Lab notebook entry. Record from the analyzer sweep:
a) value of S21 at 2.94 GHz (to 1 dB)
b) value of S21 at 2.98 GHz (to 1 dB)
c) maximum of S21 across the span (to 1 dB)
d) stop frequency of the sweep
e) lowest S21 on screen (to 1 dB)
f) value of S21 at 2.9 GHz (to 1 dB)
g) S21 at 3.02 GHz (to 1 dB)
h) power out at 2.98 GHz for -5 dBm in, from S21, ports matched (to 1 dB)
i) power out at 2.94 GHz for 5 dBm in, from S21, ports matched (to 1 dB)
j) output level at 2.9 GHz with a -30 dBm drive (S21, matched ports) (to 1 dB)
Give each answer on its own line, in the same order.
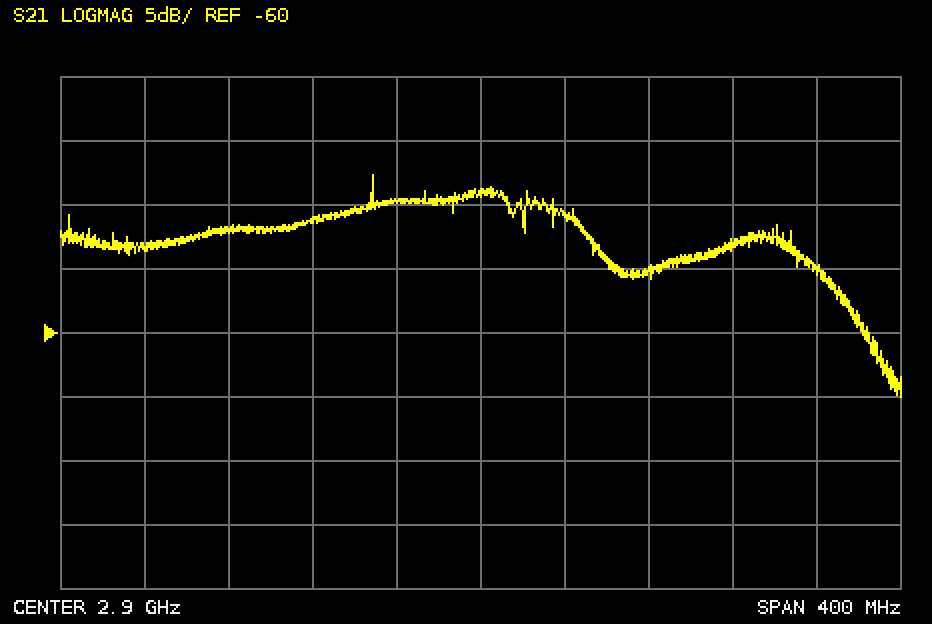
-51 dB
-55 dB
-48 dB
3.1 GHz
-65 dB
-49 dB
-53 dB
-60 dBm
-46 dBm
-79 dBm
